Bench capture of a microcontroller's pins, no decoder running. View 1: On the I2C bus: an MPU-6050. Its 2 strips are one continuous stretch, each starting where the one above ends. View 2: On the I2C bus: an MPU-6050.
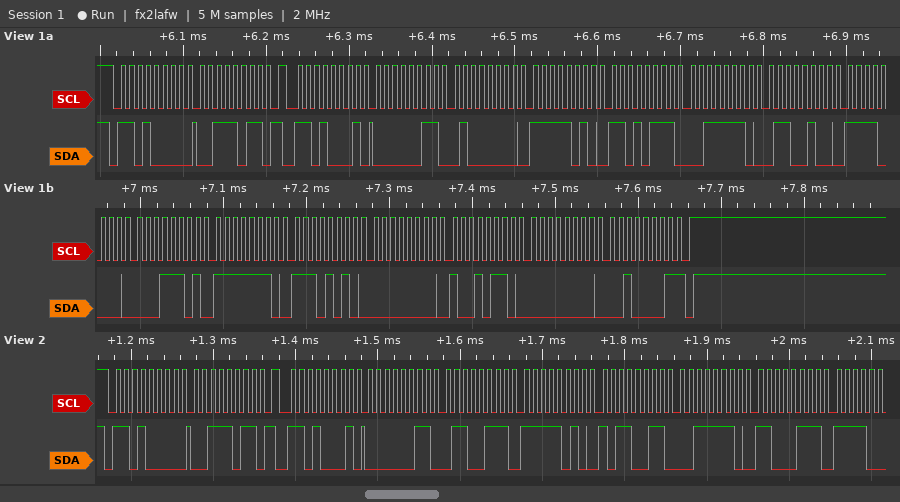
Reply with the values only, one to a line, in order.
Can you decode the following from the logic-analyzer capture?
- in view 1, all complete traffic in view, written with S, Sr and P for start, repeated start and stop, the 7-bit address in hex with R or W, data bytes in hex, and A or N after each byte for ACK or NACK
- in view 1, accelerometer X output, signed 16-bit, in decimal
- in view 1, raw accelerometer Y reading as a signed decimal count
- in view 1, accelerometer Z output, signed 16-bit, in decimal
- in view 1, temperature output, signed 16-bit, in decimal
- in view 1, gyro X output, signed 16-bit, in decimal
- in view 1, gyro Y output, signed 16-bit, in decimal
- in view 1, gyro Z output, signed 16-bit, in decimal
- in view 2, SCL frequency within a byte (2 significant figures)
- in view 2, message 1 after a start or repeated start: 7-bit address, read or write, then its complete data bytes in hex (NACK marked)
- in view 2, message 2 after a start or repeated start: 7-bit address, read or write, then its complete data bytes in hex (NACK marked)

S 68W A 3B A Sr 68R A 03 A 40 A FA A D7 A 3E A 64 A F0 A 1D A FE A EA A 00 A 96 A 00 A 21 N P
832
-1321
15972
-4067
-278
150
33
100 kHz
0x68 write: 3B
0x68 read: 03 67 FA B3 3E C7
